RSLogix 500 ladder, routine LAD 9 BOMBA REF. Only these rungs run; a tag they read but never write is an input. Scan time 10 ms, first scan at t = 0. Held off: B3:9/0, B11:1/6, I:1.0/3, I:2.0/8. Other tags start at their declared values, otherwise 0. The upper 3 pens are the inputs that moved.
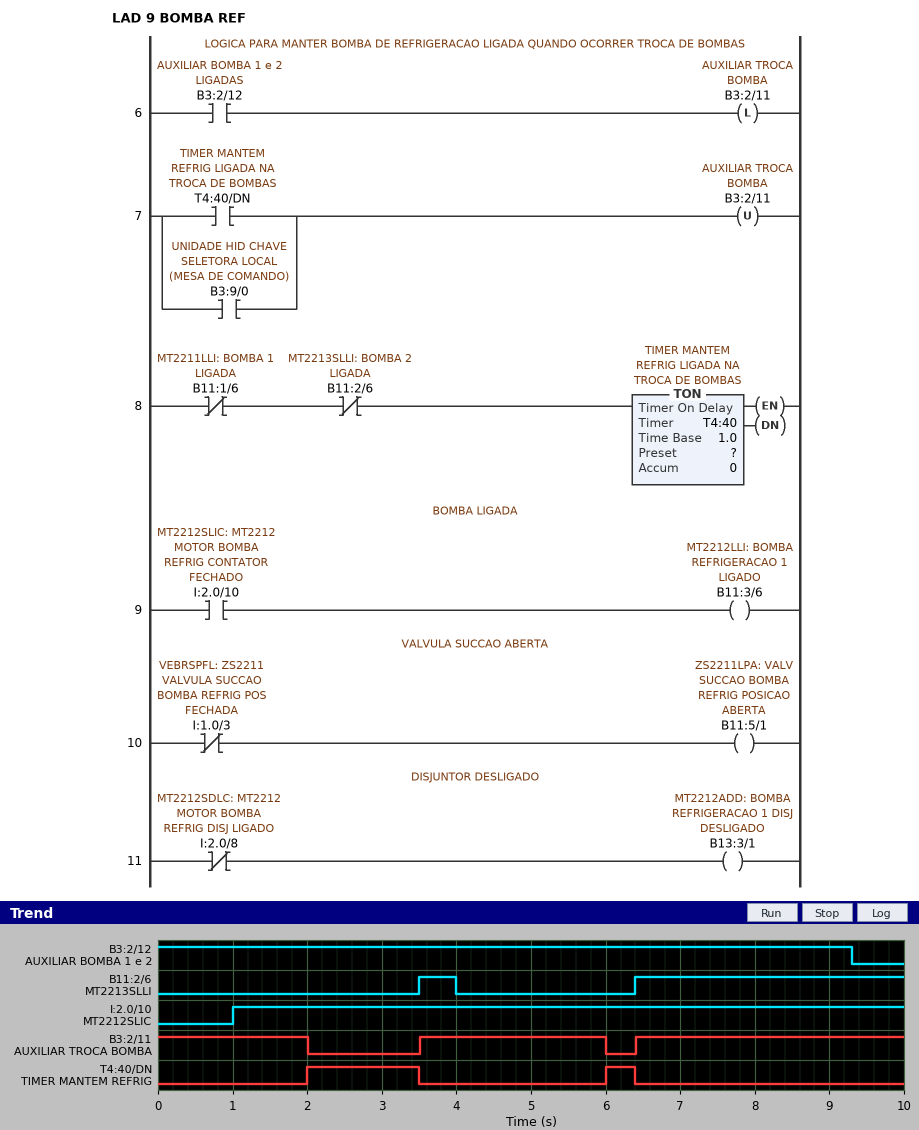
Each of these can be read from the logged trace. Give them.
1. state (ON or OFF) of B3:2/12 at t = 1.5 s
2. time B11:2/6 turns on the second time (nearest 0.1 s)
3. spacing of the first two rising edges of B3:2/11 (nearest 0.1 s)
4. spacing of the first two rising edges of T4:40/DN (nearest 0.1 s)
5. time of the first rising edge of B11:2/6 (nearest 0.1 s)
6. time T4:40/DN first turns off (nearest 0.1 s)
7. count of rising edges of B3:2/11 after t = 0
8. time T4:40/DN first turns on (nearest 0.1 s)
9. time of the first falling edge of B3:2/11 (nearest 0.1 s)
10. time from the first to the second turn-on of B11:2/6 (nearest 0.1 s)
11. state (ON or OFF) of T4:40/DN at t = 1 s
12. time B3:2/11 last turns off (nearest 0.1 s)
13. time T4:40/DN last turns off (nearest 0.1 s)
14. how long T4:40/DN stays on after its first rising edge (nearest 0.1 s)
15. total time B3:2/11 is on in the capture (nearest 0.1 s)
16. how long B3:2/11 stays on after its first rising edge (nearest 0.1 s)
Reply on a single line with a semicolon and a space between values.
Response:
ON; 6.4 s; 2.9 s; 4.0 s; 3.5 s; 3.5 s; 2; 2.0 s; 2.0 s; 2.9 s; OFF; 6.0 s; 6.4 s; 1.5 s; 8.1 s; 2.5 s
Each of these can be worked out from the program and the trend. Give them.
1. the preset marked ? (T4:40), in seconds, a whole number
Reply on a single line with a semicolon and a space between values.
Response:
2 s
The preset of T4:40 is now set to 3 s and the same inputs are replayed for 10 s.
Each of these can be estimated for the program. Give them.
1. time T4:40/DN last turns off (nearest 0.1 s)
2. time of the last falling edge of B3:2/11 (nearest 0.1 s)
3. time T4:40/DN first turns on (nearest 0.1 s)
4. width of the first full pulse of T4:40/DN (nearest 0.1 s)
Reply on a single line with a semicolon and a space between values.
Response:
3.5 s; 3.0 s; 3.0 s; 0.5 s
